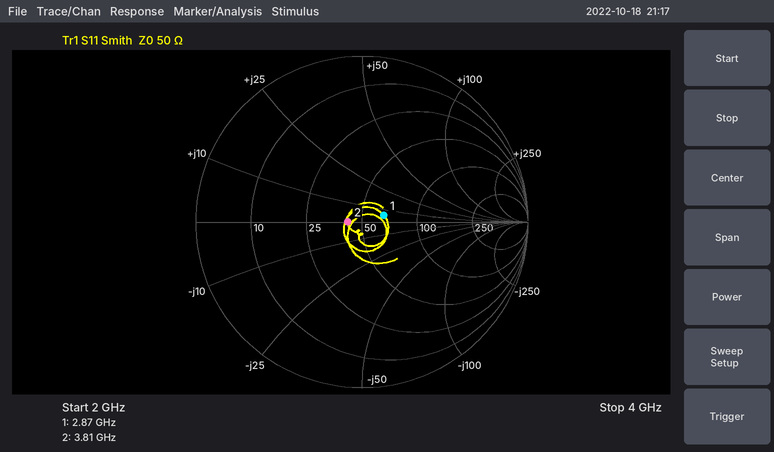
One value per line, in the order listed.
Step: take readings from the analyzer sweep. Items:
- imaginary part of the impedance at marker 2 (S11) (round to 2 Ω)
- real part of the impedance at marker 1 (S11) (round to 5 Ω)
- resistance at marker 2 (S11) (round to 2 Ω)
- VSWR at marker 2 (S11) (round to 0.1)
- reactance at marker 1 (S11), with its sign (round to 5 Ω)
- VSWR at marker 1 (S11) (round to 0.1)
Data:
0 Ω
65 Ω
42 Ω
1.2
+5 Ω
1.3
